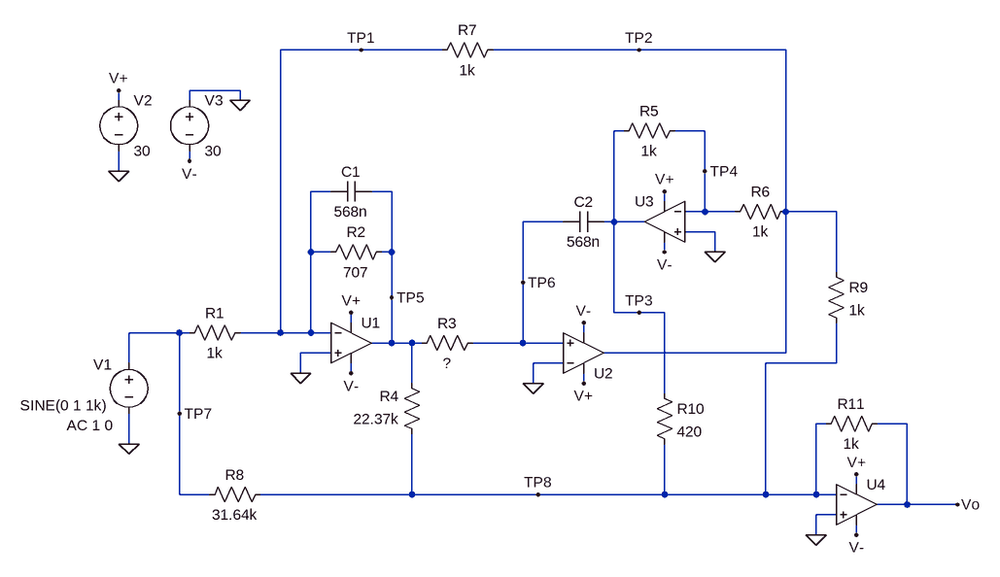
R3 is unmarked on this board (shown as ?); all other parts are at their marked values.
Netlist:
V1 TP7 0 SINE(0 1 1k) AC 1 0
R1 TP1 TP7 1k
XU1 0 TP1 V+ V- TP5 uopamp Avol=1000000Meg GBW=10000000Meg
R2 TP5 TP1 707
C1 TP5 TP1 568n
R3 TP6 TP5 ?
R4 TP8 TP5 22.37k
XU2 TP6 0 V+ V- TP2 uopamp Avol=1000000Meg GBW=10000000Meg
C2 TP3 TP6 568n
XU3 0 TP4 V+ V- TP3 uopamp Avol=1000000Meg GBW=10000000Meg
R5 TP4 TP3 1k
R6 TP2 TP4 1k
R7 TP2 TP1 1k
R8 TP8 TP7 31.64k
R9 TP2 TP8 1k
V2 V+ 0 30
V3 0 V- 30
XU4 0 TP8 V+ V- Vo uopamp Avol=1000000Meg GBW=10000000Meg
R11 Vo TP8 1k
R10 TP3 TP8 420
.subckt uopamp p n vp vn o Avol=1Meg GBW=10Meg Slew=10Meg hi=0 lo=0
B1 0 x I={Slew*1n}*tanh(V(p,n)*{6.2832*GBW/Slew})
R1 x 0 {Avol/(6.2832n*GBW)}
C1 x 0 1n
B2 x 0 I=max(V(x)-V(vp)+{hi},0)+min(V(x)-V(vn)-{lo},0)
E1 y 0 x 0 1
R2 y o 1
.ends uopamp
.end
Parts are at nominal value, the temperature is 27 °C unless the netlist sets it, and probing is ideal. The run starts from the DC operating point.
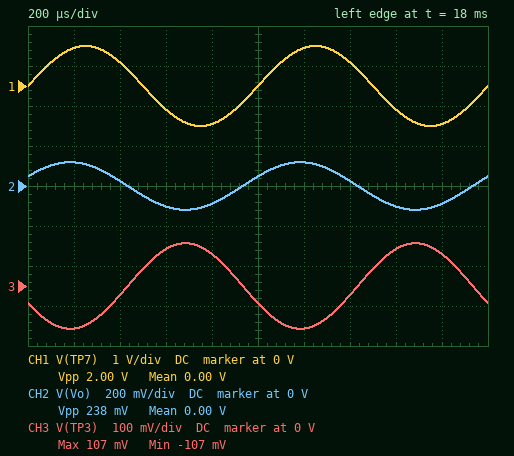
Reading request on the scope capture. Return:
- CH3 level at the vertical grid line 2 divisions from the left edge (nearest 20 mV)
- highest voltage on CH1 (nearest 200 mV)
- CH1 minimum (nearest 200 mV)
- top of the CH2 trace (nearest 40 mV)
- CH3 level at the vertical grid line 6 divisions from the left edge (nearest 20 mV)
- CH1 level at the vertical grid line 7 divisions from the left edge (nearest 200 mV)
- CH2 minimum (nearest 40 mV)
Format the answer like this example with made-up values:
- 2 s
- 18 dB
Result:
- -20 mV
- 1.0 V
- -1.0 V
- 120 mV
- -100 mV
- 600 mV
- -120 mV
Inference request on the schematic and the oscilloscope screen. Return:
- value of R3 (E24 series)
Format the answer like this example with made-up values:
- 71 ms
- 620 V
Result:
- 750 Ω
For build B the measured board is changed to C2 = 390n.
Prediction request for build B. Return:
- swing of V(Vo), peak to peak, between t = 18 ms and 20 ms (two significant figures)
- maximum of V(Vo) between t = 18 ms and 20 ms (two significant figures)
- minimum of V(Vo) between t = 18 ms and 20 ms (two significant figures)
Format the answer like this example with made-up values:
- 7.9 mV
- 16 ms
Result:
- 390 mV
- 200 mV
- -200 mV
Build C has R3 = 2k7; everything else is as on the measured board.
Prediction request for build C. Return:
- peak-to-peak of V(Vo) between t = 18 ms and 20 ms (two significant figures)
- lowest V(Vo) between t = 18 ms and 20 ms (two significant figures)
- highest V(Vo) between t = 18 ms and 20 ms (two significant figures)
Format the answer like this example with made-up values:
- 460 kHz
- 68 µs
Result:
- 18 mV
- -9.0 mV
- 9.0 mV
